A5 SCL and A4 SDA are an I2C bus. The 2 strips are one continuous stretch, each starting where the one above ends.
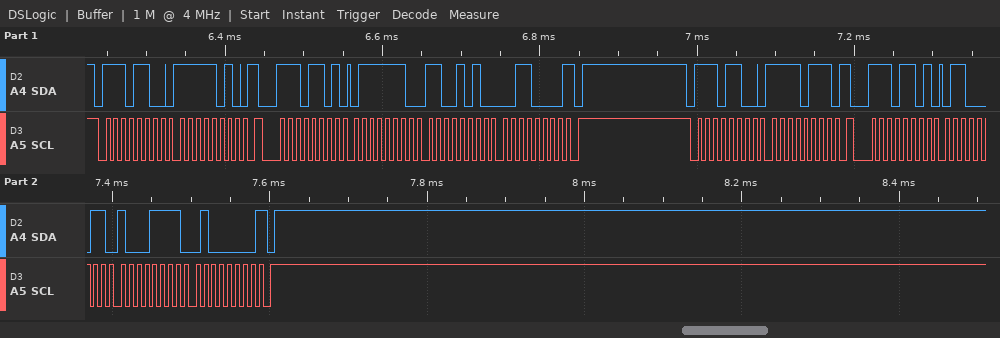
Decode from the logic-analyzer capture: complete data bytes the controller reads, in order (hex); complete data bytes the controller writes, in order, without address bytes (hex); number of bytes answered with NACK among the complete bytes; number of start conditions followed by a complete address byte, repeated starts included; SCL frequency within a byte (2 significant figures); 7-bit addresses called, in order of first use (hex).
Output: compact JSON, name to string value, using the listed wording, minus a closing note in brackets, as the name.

{"complete data bytes the controller reads, in order": "7E CA 30 63 8F 40", "complete data bytes the controller writes, in order, without address bytes": "FA F7", "number of bytes answered with NACK among the complete bytes": "2", "number of start conditions followed by a complete address byte, repeated starts included": "4", "SCL frequency within a byte": "100 kHz", "7-bit addresses called, in order of first use": "0x76"}
